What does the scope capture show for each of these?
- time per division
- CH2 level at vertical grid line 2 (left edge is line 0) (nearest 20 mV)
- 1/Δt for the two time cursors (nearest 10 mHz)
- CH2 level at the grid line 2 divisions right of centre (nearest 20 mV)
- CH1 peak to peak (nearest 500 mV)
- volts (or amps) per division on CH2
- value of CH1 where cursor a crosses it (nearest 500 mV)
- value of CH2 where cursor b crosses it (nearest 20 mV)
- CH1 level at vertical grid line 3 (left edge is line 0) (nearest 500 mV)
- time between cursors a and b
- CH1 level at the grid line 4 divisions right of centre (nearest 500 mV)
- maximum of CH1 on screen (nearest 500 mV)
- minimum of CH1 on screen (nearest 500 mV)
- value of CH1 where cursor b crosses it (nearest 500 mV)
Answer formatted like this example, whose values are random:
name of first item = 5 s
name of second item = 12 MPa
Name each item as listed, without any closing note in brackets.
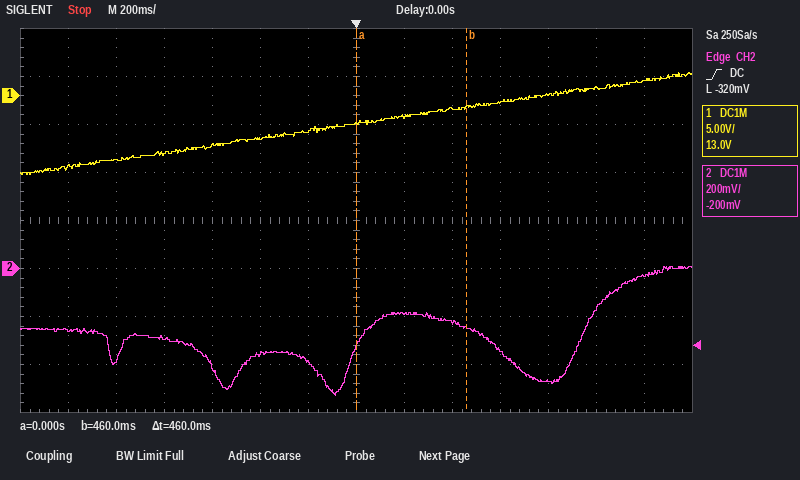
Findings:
time per division = 200 ms
CH2 level at vertical grid line 2 (left edge is line 0) = -380 mV
1/Δt for the two time cursors = 2.17 Hz
CH2 level at the grid line 2 divisions right of centre = -220 mV
CH1 peak to peak = 10.5 V
volts (or amps) per division on CH2 = 200 mV
value of CH1 where cursor a crosses it = -3.0 V
value of CH2 where cursor b crosses it = -240 mV
CH1 level at vertical grid line 3 (left edge is line 0) = -6.0 V
time between cursors a and b = 460 ms
CH1 level at the grid line 4 divisions right of centre = 0.0 V
maximum of CH1 on screen = 2.5 V
minimum of CH1 on screen = -8.0 V
value of CH1 where cursor b crosses it = -1.0 V
